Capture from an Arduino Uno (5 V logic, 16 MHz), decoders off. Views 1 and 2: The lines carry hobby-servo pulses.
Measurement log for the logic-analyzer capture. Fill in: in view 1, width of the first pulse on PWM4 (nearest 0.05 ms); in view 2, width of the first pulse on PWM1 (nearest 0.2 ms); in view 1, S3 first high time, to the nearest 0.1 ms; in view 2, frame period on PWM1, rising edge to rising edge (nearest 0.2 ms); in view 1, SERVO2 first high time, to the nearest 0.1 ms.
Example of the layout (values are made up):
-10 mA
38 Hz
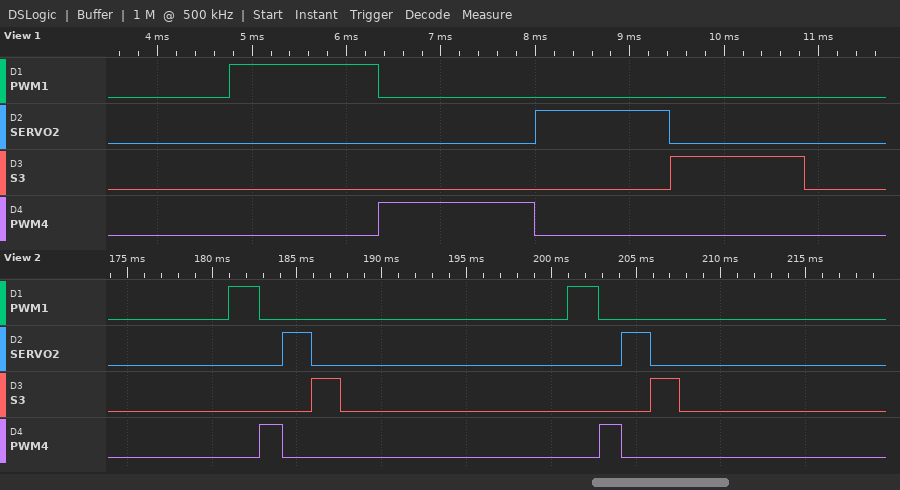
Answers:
1.65 ms
1.8 ms
1.4 ms
20.0 ms
1.4 ms
